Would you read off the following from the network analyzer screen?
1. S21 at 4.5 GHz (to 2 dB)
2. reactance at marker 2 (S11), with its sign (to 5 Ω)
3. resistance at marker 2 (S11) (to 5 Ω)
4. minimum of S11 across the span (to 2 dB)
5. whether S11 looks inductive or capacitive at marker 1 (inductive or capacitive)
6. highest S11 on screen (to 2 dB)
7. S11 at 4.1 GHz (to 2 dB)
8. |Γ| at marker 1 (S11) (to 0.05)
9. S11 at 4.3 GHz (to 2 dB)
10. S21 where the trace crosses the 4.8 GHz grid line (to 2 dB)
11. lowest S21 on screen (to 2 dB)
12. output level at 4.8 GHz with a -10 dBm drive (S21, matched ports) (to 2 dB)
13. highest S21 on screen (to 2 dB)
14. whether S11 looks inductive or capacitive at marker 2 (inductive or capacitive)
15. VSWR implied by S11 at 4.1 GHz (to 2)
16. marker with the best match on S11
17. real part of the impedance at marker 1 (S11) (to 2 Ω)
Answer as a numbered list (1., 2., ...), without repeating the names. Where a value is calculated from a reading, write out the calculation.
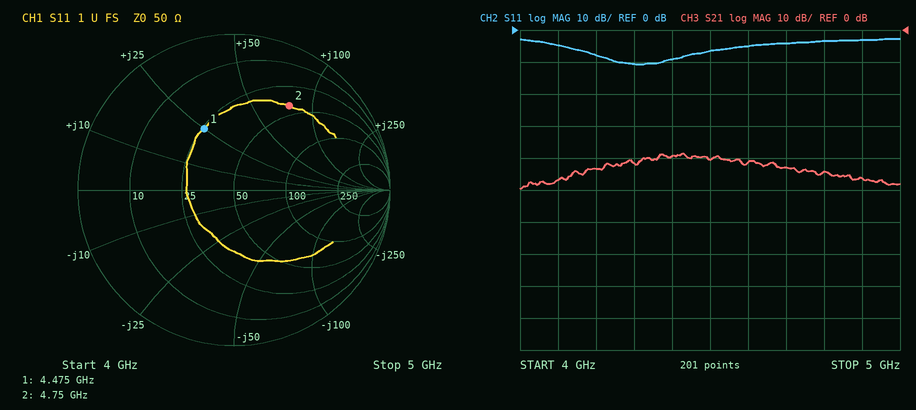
1. -40 dB
2. +75 Ω
3. 40 Ω
4. -10 dB
5. inductive
6. -2 dB
7. -4 dB
8. 0.45
9. -10 dB
10. -44 dB
11. -50 dB
12. -10 dBm + (-44 dB) = -54 dBm
13. -38 dB
14. inductive
15. |Γ| = 10^(-4/20) = 0.6310; VSWR = (1 + 0.6310)/(1 − 0.6310) ≈ 4
16. marker 1
17. 26 Ω
